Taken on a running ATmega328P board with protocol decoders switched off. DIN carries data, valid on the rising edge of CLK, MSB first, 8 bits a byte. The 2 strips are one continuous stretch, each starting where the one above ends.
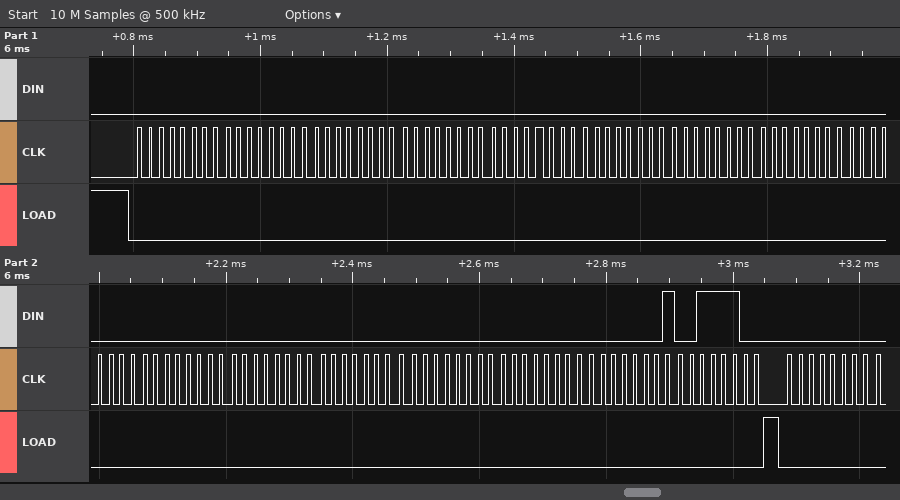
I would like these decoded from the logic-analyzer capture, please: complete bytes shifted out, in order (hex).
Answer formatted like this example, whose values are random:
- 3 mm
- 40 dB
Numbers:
- 0x00 0x00 0x00 0x00 0x00 0x00 0x00 0x00 0x00 0x00 0x00 0x00 0x00 0x00 0x01 0x3C 0x00
